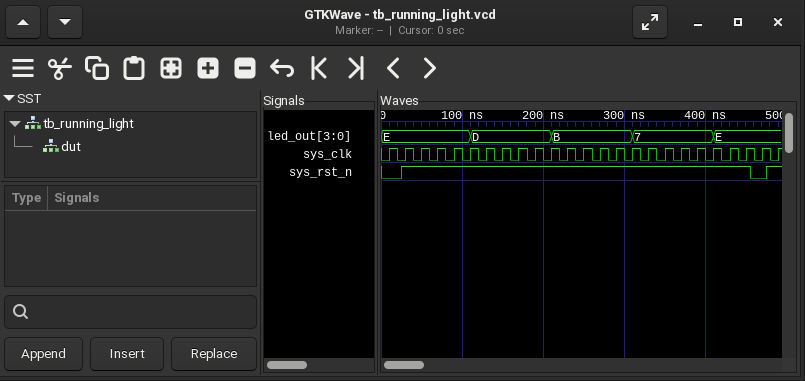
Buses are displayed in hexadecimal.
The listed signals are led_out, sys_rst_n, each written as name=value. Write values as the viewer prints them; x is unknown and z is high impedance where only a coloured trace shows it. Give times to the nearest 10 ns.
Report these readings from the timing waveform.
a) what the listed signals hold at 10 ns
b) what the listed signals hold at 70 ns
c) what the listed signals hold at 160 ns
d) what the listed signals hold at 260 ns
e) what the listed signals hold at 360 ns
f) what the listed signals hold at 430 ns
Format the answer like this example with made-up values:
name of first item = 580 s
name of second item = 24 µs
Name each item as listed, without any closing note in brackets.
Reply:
what the listed signals hold at 10 ns = led_out=E, sys_rst_n=0
what the listed signals hold at 70 ns = led_out=E, sys_rst_n=1
what the listed signals hold at 160 ns = led_out=D, sys_rst_n=1
what the listed signals hold at 260 ns = led_out=B, sys_rst_n=1
what the listed signals hold at 360 ns = led_out=7, sys_rst_n=1
what the listed signals hold at 430 ns = led_out=E, sys_rst_n=1
